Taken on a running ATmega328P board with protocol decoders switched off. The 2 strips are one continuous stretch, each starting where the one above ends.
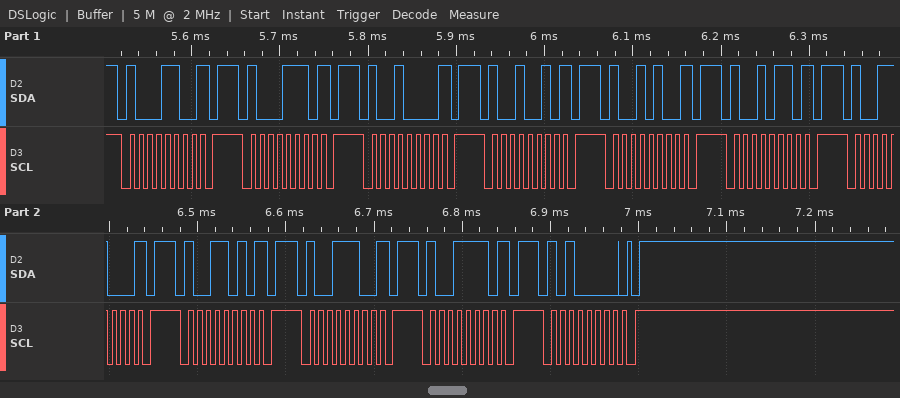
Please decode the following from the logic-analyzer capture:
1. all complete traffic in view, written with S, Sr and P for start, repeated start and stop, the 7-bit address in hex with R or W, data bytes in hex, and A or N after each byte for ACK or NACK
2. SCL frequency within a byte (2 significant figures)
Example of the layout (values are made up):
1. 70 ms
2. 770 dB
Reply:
1. S 46W N P S 47W N P S 48W N P S 49W N P S 4AW N P S 4BW N P S 4CW N P S 4DW N P S 4EW N P S 4FW N P S 50W A P
2. 100 kHz
